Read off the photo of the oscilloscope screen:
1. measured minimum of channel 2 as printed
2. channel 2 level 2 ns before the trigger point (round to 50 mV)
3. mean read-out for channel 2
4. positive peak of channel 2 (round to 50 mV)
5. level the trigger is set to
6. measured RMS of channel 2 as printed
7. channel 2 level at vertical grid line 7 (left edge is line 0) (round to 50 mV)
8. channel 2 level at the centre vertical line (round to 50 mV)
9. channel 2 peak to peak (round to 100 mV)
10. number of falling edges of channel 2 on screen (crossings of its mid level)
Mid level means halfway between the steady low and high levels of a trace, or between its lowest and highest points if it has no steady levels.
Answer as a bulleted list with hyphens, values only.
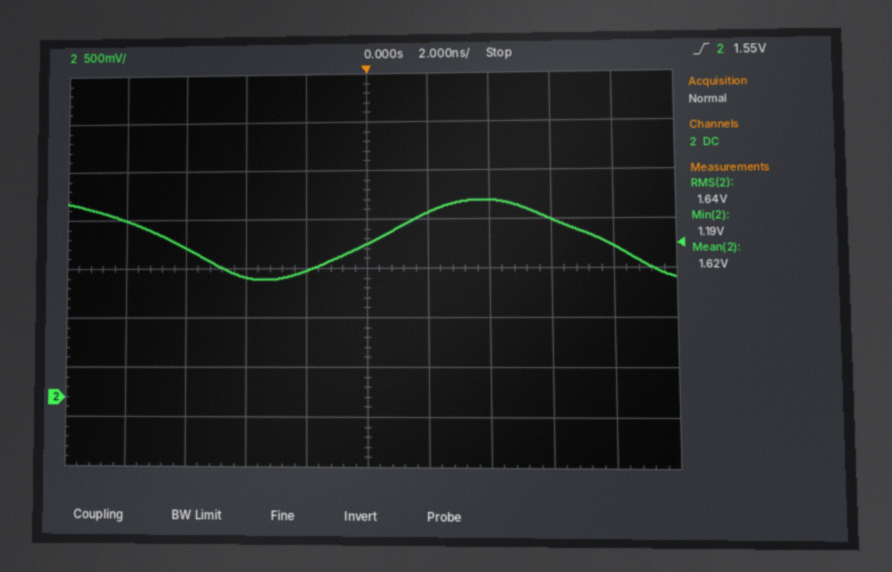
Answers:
- 1.19 V
- 1.30 V
- 1.62 V
- 2.00 V
- 1.55 V
- 1.64 V
- 2.00 V
- 1.55 V
- 800 mV
- 2
